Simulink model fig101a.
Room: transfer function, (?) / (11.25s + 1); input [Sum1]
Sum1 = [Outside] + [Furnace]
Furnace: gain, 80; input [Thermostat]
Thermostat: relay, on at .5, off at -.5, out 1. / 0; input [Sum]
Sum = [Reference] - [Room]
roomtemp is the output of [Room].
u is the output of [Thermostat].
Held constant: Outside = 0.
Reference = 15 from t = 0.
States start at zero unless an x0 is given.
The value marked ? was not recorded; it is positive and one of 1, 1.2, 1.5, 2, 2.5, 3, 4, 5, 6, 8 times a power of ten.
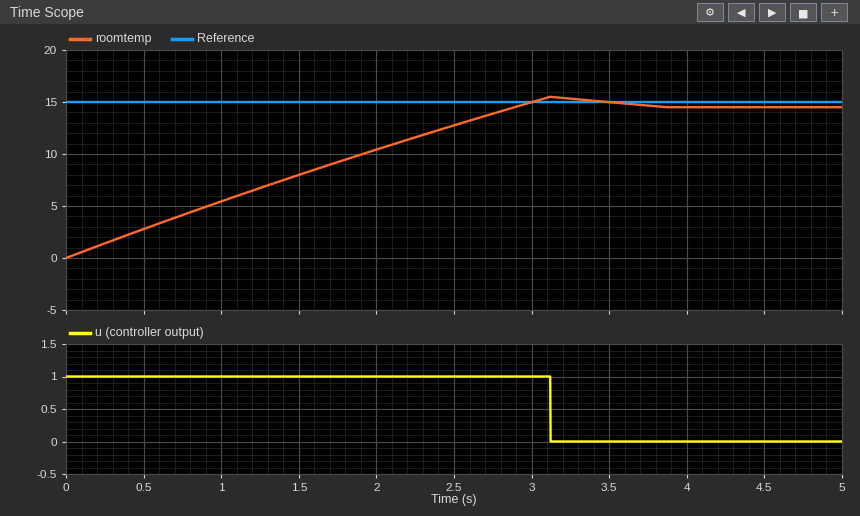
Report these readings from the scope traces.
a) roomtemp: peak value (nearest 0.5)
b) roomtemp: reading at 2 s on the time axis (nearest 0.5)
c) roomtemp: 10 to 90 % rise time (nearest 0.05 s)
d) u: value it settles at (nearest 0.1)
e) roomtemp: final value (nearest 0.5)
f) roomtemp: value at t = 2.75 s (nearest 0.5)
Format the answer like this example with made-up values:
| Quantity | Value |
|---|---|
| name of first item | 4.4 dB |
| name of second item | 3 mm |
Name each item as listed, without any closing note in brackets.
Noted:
| Quantity | Value |
|---|---|
| roomtemp: peak value | 15.5 |
| roomtemp: reading at 2 s on the time axis | 10.5 |
| roomtemp: 10 to 90 % rise time | 2.30 s |
| u: value it settles at | 0.0 |
| roomtemp: final value | 14.5 |
| roomtemp: value at t = 2.75 s | 14.0 |
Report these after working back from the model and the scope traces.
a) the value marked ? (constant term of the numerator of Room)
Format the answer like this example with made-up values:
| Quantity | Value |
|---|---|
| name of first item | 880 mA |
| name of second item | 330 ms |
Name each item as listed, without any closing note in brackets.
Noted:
| Quantity | Value |
|---|---|
| the value marked ? | 0.8 |
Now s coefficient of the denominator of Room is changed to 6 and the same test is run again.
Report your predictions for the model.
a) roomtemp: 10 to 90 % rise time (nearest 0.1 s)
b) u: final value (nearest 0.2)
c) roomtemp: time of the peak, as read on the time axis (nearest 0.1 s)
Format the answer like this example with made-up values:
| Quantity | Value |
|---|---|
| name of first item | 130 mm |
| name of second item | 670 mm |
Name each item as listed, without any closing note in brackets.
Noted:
| Quantity | Value |
|---|---|
| roomtemp: 10 to 90 % rise time | 1.2 s |
| u: final value | 0.0 |
| roomtemp: time of the peak, as read on the time axis | 1.7 s |
